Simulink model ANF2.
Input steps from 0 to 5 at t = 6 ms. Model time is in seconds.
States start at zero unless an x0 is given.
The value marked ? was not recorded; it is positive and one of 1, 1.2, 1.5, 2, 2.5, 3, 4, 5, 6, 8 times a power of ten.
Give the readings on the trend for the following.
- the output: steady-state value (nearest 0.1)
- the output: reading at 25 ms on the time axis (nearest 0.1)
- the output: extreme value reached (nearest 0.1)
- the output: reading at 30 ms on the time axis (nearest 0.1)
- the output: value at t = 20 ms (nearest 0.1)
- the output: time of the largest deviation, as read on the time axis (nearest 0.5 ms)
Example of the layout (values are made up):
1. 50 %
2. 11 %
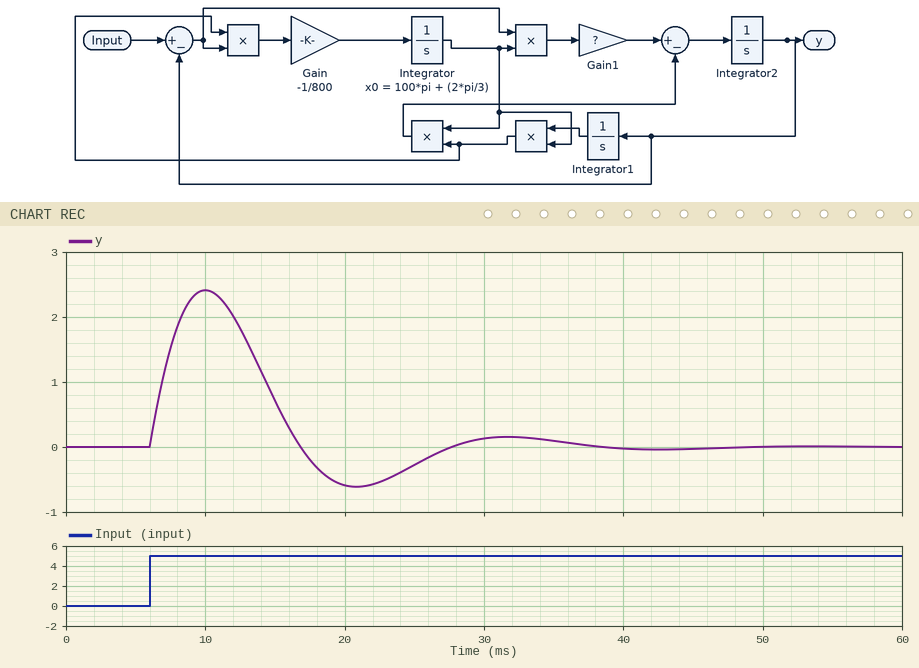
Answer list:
1. 0.0
2. -0.3
3. 2.4
4. 0.1
5. -0.6
6. 10.0 ms
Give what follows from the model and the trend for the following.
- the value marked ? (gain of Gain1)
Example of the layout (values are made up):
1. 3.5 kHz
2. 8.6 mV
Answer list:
1. 0.8
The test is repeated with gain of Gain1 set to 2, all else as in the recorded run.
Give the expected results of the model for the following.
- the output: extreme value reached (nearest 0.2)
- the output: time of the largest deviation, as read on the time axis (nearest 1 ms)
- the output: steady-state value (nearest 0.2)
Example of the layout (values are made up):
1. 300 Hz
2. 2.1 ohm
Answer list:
1. 3.6
2. 9 ms
3. 0.0
